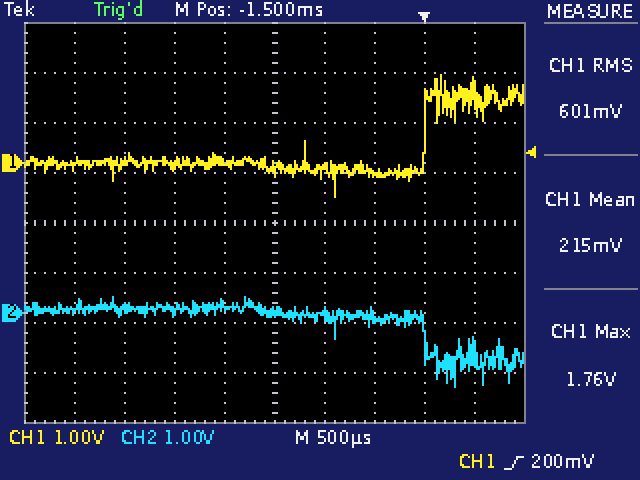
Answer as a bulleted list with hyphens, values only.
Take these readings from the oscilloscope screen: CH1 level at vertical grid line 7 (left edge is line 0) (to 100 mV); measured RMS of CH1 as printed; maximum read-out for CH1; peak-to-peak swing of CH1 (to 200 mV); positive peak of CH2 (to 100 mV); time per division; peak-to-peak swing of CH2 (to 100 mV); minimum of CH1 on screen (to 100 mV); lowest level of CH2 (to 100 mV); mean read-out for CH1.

- -200 mV
- 601 mV
- 1.76 V
- 2.4 V
- 300 mV
- 500 µs
- 1.8 V
- -700 mV
- -1.5 V
- 215 mV
